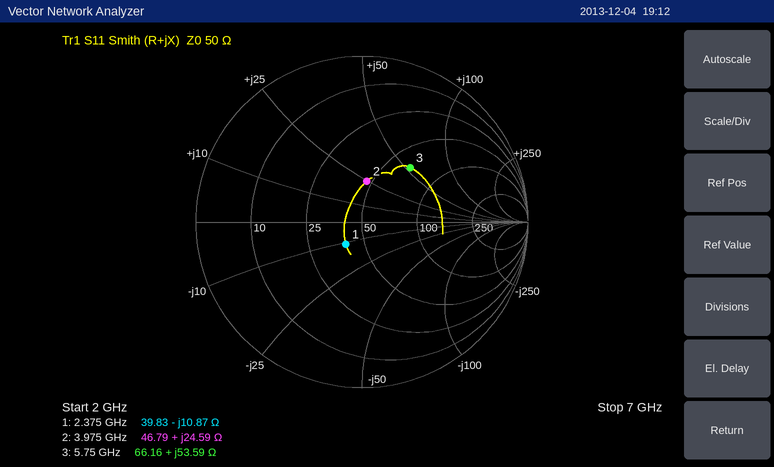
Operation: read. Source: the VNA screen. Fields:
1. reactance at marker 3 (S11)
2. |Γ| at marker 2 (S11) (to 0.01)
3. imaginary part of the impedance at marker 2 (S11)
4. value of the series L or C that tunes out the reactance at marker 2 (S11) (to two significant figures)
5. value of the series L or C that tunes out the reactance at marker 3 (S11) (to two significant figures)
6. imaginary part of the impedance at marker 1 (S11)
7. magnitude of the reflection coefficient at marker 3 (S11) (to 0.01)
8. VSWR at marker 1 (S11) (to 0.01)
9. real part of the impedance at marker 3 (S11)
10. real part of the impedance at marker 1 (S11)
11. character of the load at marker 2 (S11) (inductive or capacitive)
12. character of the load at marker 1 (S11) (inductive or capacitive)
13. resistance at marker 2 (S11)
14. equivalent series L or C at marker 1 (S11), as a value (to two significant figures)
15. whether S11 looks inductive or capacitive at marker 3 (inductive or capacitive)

+53.59 Ω
0.25
+24.59 Ω
1.6 pF
520 fF
-10.87 Ω
0.44
1.39
66.16 Ω
39.83 Ω
inductive
capacitive
46.79 Ω
6.2 pF
inductive
